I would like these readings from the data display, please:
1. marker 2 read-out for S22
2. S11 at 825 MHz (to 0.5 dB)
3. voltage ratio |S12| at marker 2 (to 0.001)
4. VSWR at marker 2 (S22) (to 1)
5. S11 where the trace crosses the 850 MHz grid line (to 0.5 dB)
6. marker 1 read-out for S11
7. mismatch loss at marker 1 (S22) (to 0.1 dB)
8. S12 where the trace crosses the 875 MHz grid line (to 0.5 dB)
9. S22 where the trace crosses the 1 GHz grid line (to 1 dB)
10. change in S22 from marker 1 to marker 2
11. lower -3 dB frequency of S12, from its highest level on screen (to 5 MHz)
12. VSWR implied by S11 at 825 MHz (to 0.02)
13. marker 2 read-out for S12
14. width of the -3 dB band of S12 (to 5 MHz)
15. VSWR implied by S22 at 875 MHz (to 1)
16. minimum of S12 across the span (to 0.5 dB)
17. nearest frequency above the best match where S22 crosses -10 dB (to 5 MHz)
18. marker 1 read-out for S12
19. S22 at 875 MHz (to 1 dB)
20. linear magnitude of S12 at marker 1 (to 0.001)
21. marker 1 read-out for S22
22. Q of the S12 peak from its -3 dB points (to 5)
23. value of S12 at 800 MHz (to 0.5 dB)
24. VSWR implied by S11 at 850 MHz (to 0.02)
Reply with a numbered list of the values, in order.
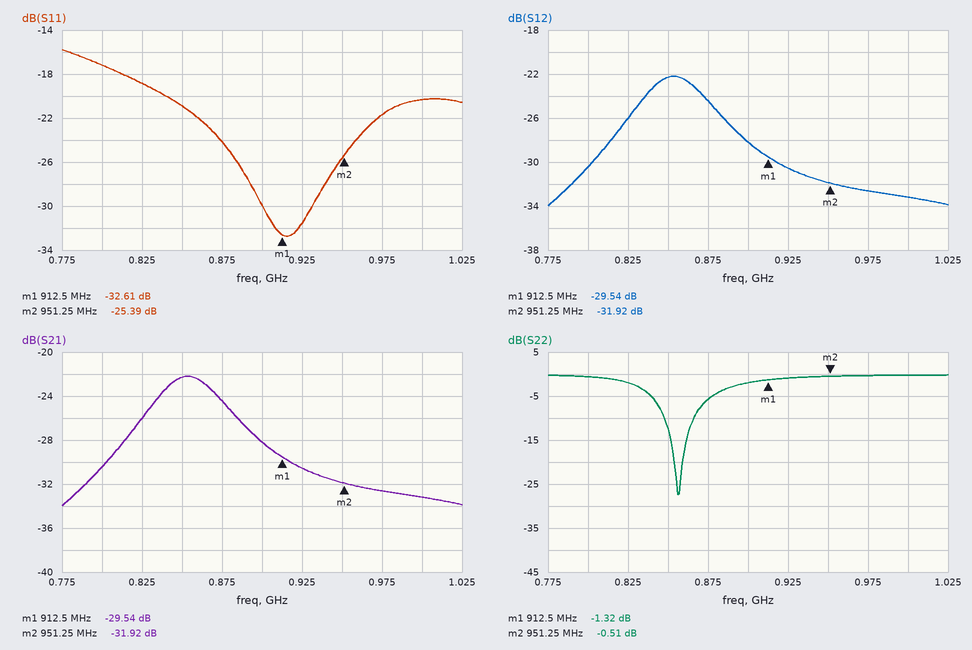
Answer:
1. -0.51 dB
2. -19.0 dB
3. 0.025
4. 34
5. -21.0 dB
6. -32.61 dB
7. 5.8 dB
8. -24.5 dB
9. 0 dB
10. 0.81 dB
11. 830 MHz
12. 1.26
13. -31.92 dB
14. 50 MHz
15. 3
16. -34.0 dB
17. 865 MHz
18. -29.54 dB
19. -6 dB
20. 0.033
21. -1.32 dB
22. 15
23. -30.5 dB
24. 1.20
